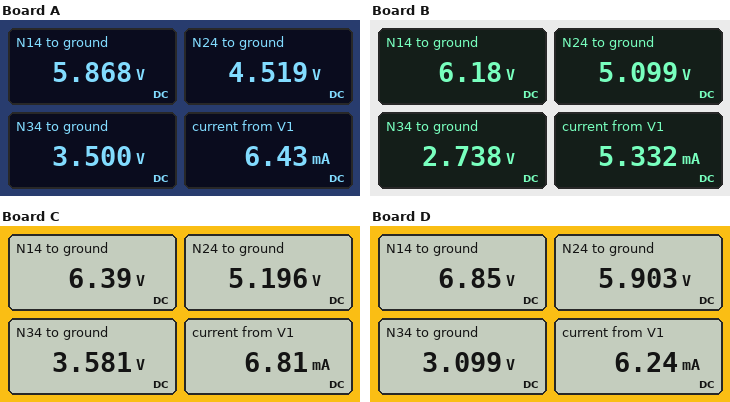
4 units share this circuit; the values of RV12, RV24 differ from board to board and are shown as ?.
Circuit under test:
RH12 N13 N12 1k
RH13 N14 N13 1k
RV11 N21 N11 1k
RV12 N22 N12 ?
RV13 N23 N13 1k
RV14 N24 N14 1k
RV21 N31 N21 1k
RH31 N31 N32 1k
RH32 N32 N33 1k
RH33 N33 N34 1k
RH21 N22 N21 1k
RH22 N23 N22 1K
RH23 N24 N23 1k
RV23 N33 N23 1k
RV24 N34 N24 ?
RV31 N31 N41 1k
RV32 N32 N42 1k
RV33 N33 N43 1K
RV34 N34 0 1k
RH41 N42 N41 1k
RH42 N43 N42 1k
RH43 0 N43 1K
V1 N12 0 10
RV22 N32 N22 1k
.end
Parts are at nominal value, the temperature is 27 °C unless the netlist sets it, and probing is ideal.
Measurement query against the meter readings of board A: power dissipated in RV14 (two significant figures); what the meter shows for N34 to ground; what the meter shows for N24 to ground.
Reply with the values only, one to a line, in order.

1.8 mW
3.500 V
4.519 V
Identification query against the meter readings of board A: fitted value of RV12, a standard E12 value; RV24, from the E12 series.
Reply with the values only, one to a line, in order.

820 Ω
390 Ω
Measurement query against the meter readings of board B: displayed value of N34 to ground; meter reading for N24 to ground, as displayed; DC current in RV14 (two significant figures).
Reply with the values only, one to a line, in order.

2.738 V
5.099 V
1.1 mA
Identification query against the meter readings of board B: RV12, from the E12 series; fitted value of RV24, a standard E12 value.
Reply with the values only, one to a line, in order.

1.5 kΩ
1.5 kΩ
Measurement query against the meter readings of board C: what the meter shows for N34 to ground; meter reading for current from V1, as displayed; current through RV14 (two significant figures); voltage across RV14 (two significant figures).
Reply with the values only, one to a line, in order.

3.581 V
6.81 mA
1.2 mA
1.2 V
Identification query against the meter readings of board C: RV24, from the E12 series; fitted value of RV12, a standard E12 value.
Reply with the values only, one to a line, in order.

680 Ω
470 Ω
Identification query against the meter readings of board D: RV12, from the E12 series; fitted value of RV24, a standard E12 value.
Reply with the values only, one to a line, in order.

560 Ω
1.8 kΩ
